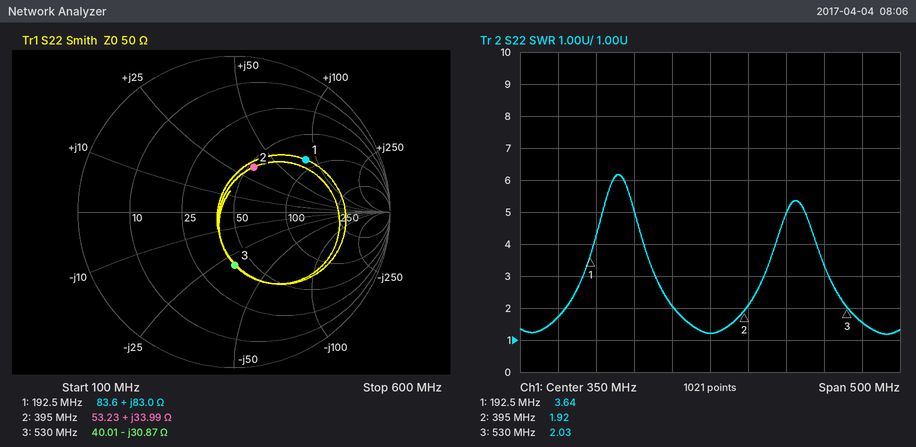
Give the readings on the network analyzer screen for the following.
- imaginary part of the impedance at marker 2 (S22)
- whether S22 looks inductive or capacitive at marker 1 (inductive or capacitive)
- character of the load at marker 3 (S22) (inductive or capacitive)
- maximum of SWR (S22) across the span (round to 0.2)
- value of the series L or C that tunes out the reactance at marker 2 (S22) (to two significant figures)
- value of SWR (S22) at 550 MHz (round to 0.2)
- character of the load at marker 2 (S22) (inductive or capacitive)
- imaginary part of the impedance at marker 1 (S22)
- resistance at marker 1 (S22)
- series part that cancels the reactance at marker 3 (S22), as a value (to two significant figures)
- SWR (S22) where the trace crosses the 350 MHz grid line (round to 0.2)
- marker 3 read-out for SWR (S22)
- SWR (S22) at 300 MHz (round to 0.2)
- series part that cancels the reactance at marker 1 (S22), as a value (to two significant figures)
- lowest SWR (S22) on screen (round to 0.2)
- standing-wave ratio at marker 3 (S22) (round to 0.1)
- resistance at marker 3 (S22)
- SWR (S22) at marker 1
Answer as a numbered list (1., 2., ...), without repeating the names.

1. +33.99 Ω
2. inductive
3. capacitive
4. 6.2
5. 12 pF
6. 1.6
7. inductive
8. +83.0 Ω
9. 83.6 Ω
10. 9.3 nH
11. 1.2
12. 2.03
13. 2.0
14. 10.0 pF
15. 1.2
16. 2.0
17. 40.01 Ω
18. 3.64
